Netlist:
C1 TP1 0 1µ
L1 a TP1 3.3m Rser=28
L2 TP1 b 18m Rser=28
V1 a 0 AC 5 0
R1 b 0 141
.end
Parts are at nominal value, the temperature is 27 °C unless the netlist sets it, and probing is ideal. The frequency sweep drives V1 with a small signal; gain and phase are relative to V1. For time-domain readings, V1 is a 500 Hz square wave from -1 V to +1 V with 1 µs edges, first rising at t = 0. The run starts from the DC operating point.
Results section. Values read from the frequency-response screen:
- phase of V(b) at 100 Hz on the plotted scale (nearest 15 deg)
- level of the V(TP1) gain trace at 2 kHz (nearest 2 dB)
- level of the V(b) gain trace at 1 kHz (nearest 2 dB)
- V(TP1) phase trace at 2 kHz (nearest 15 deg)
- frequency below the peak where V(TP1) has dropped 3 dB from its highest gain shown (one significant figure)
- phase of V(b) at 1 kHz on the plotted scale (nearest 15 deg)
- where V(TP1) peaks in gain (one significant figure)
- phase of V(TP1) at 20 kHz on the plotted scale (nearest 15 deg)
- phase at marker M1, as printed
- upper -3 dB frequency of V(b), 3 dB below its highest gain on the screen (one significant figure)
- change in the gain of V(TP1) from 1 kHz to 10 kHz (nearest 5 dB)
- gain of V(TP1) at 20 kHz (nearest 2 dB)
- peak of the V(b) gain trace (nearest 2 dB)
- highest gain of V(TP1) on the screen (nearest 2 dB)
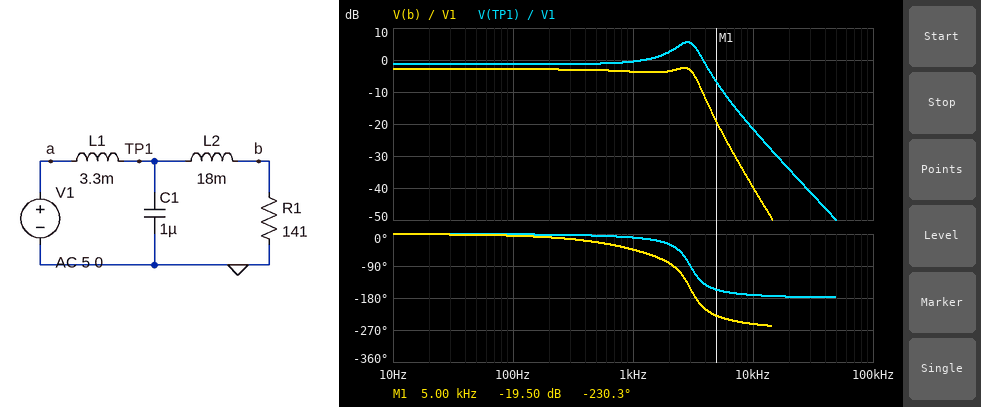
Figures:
0 deg
2 dB
-4 dB
-30 deg
2 kHz
-45 deg
3 kHz
-180 deg
-230.3 deg
3 kHz
-20 dB
-34 dB
-2 dB
6 dB
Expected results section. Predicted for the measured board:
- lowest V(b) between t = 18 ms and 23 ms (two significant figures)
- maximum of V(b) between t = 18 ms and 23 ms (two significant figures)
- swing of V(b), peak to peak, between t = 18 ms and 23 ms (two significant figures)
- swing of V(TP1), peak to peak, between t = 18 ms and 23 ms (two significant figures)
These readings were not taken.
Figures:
-820 mV
820 mV
1.6 V
3.3 V
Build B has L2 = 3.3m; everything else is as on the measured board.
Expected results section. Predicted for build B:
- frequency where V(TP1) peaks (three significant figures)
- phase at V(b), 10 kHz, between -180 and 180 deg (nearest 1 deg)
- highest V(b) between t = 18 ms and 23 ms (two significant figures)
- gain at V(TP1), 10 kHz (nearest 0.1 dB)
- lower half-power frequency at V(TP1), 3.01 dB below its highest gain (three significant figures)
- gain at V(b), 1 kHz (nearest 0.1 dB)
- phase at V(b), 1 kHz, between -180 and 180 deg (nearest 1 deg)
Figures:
2.73 kHz
140 deg
1.1 V
-21.3 dB
841 Hz
-2.3 dB
-22 deg
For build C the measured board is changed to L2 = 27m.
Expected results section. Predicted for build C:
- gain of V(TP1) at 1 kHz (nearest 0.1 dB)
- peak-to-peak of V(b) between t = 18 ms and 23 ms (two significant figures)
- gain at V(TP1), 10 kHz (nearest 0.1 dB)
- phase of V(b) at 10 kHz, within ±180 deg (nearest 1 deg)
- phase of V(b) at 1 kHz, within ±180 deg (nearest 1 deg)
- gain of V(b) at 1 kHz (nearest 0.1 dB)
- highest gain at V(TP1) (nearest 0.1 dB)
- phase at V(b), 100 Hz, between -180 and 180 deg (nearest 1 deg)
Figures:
-0.2 dB
1.5 V
-21.6 dB
104 deg
-54 deg
-4.8 dB
6.2 dB
-6 deg
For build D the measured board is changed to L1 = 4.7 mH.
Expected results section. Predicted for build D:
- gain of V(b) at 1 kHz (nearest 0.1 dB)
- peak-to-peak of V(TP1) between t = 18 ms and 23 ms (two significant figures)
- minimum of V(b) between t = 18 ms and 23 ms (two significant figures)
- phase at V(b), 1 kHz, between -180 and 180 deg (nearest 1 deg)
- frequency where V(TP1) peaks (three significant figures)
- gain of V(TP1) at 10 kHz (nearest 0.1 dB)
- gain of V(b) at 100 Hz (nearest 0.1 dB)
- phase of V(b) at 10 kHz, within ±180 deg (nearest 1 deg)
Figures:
-3.5 dB
3.4 V
-910 mV
-46 deg
2.49 kHz
-24.8 dB
-2.9 dB
104 deg
